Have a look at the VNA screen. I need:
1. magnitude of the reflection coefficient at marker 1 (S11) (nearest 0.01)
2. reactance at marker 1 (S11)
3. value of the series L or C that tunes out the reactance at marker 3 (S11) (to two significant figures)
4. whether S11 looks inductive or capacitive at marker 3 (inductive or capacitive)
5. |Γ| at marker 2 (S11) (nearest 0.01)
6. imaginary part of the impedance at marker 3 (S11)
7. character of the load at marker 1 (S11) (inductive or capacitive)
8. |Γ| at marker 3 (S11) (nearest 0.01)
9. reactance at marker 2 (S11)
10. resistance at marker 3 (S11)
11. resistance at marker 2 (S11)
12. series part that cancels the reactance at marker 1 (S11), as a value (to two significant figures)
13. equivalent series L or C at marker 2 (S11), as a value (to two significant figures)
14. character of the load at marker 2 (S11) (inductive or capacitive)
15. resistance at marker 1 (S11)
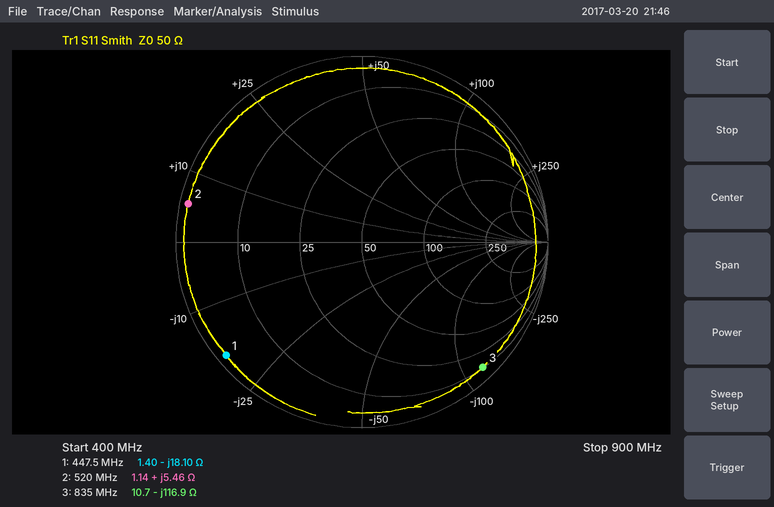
0.95
-18.10 Ω
22 nH
capacitive
0.96
-116.9 Ω
capacitive
0.94
+5.46 Ω
10.7 Ω
1.14 Ω
6.4 nH
1.7 nH
inductive
1.40 Ω
